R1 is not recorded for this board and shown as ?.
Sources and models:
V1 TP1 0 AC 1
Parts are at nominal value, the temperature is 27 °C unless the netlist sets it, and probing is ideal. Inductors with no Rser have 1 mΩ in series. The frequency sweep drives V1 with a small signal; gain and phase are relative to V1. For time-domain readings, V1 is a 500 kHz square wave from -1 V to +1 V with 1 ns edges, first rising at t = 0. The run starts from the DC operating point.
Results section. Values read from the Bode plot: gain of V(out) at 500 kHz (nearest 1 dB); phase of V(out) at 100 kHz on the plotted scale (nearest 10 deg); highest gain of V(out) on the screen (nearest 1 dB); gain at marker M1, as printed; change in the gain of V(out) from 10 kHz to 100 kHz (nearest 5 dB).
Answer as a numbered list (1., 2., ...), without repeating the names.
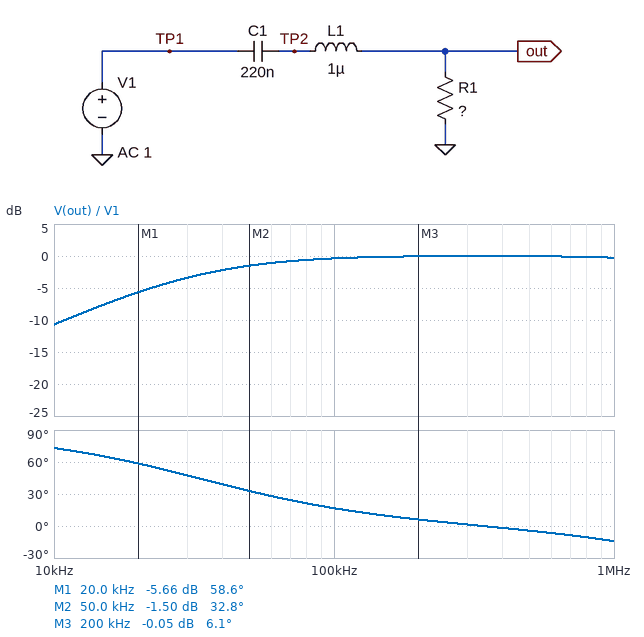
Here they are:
1. 0 dB
2. 20 deg
3. 0 dB
4. -5.66 dB
5. 10 dB
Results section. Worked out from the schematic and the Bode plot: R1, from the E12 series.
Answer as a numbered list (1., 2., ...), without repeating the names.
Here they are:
1. 22 Ω
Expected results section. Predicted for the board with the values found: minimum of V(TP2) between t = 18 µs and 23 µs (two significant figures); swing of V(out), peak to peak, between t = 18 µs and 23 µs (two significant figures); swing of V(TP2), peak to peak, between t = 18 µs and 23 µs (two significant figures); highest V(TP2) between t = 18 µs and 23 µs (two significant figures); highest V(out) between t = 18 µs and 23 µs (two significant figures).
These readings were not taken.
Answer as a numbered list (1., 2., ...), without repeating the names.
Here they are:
1. -1.1 V
2. 2.1 V
3. 2.2 V
4. 1.1 V
5. 1.1 V
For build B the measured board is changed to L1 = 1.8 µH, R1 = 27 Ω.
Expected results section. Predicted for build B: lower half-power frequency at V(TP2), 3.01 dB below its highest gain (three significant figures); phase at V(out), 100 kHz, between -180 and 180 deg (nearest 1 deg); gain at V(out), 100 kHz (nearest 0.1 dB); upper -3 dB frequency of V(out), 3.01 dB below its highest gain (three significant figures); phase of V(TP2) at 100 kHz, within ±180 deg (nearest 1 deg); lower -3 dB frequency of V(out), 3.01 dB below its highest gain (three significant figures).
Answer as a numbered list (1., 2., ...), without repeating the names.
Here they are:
1. 27.0 kHz
2. 13 deg
3. -0.2 dB
4. 2.41 MHz
5. 15 deg
6. 26.5 kHz
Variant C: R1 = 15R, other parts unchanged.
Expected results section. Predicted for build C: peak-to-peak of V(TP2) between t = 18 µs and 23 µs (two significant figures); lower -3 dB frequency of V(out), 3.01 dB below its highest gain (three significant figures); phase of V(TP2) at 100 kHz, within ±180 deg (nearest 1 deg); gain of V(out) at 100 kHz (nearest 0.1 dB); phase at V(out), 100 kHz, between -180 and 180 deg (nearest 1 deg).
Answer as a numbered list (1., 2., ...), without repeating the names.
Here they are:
1. 2.3 V
2. 47.3 kHz
3. 26 deg
4. -0.8 dB
5. 24 deg
